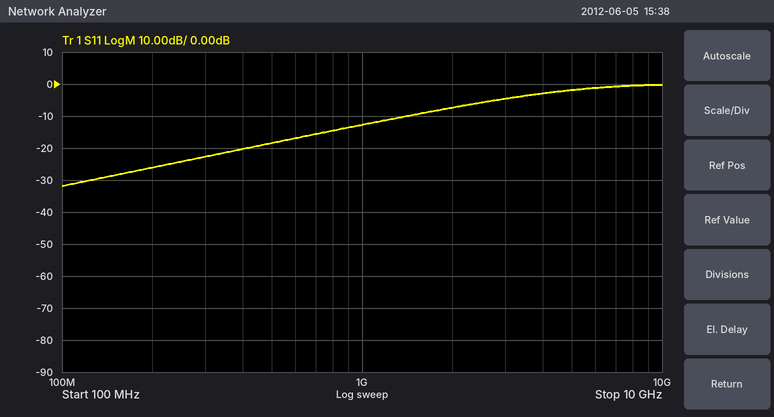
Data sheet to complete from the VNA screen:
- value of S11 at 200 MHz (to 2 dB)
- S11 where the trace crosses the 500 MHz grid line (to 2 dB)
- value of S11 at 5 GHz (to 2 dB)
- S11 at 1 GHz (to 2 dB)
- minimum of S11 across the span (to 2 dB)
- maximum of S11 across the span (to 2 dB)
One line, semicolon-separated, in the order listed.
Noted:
-26 dB; -18 dB; -2 dB; -12 dB; -32 dB; 0 dB
